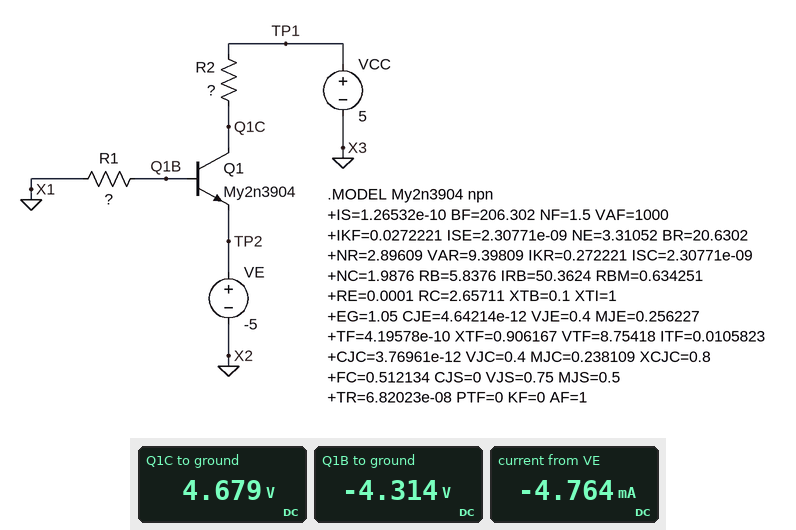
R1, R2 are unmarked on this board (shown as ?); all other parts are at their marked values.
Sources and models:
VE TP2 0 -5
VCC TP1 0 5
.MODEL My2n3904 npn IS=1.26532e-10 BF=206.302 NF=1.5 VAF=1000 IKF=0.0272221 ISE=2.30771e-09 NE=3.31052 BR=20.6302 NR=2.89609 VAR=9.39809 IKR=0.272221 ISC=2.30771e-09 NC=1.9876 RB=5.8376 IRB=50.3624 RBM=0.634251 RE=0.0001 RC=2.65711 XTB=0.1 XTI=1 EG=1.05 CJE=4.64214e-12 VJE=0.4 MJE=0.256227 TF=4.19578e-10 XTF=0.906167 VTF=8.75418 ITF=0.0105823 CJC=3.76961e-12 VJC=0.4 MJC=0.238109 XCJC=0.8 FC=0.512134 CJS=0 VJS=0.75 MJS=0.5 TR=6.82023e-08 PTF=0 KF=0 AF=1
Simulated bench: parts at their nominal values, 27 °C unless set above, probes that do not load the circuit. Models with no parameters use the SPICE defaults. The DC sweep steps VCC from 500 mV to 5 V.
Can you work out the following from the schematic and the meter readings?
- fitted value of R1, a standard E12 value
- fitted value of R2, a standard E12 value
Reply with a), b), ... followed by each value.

a) 120 kΩ
b) 68 Ω
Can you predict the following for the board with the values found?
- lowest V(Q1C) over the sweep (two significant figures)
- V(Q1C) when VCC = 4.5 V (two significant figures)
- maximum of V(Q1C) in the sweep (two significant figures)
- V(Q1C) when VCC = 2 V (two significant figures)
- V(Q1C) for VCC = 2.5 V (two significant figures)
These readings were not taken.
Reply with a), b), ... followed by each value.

a) 180 mV
b) 4.2 V
c) 4.7 V
d) 1.7 V
e) 2.2 V
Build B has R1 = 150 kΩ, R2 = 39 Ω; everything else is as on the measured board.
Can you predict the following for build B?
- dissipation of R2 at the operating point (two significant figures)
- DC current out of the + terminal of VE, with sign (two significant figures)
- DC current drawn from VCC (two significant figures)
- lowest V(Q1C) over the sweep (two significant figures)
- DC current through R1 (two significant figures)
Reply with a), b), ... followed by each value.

a) 570 µW
b) -3.8 mA
c) 3.8 mA
d) 350 mV
e) 29 µA
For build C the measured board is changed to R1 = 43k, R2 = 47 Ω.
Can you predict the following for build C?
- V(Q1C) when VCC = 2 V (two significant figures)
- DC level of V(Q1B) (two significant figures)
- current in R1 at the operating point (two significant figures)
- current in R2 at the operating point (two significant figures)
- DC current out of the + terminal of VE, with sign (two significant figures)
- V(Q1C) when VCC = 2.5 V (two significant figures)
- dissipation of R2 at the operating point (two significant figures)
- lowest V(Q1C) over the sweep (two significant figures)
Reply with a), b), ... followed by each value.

a) 1.5 V
b) -4.3 V
c) 99 µA
d) 12 mA
e) -12 mA
f) 2.0 V
g) 6.3 mW
h) -42 mV
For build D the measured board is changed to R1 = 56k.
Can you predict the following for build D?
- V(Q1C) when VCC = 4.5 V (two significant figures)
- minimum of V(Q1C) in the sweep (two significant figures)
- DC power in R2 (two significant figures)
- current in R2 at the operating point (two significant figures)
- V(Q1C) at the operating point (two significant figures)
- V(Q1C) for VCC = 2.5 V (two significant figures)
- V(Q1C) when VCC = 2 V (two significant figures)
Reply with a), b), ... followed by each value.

a) 3.9 V
b) -130 mV
c) 5.9 mW
d) 9.3 mA
e) 4.4 V
f) 1.9 V
g) 1.4 V
